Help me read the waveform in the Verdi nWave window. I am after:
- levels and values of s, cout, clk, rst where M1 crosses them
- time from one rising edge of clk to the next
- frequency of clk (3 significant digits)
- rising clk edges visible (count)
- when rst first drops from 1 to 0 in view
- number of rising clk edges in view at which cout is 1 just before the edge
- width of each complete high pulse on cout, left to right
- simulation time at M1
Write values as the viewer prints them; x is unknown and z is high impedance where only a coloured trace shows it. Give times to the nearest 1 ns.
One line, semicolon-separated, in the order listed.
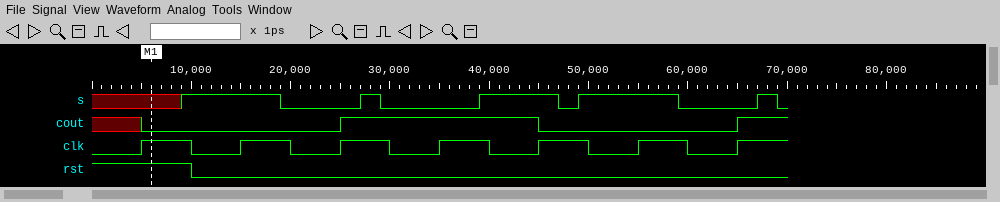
s=x, cout=0, clk=1, rst=1; 10 ns; 100 MHz; 7; 10 ns; 2; 20 ns; 6 ns
